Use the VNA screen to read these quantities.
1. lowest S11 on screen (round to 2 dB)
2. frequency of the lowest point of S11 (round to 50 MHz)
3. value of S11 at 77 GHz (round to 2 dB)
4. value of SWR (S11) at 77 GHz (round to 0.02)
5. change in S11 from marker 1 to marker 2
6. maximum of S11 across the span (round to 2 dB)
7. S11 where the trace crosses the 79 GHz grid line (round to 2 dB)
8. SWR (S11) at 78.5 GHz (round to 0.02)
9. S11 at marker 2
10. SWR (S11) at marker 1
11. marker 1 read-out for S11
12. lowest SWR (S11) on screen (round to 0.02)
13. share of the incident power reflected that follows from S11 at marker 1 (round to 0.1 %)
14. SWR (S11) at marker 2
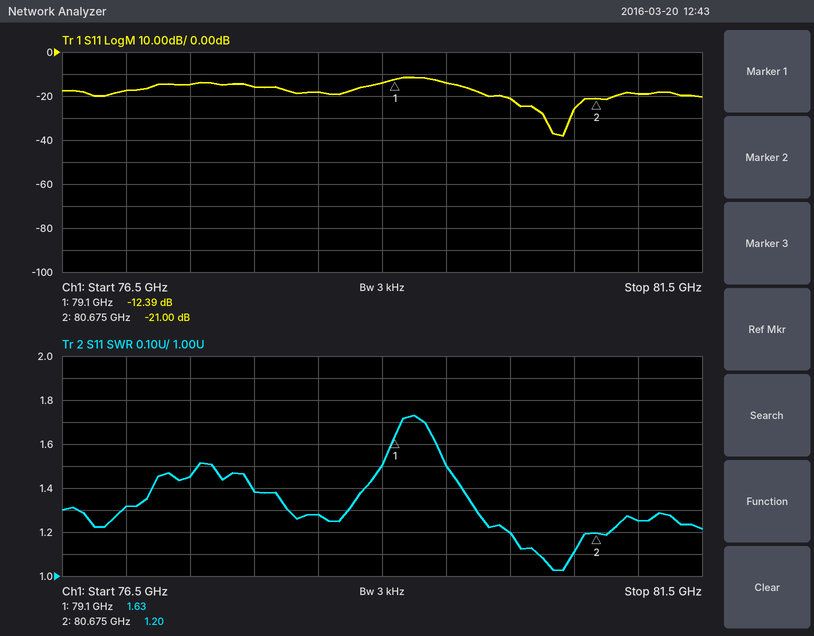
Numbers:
-38 dB
80.40 GHz
-18 dB
1.32
-8.61 dB
-12 dB
-14 dB
1.28
-21.00 dB
1.63
-12.39 dB
1.02
5.8 %
1.20
